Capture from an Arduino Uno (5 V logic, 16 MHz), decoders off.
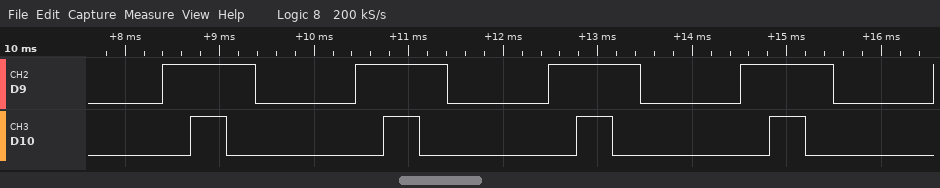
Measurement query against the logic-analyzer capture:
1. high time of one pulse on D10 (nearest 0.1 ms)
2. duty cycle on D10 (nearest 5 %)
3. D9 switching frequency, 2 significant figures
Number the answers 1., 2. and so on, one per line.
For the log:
1. 0.4 ms
2. 20 %
3. 490 Hz
